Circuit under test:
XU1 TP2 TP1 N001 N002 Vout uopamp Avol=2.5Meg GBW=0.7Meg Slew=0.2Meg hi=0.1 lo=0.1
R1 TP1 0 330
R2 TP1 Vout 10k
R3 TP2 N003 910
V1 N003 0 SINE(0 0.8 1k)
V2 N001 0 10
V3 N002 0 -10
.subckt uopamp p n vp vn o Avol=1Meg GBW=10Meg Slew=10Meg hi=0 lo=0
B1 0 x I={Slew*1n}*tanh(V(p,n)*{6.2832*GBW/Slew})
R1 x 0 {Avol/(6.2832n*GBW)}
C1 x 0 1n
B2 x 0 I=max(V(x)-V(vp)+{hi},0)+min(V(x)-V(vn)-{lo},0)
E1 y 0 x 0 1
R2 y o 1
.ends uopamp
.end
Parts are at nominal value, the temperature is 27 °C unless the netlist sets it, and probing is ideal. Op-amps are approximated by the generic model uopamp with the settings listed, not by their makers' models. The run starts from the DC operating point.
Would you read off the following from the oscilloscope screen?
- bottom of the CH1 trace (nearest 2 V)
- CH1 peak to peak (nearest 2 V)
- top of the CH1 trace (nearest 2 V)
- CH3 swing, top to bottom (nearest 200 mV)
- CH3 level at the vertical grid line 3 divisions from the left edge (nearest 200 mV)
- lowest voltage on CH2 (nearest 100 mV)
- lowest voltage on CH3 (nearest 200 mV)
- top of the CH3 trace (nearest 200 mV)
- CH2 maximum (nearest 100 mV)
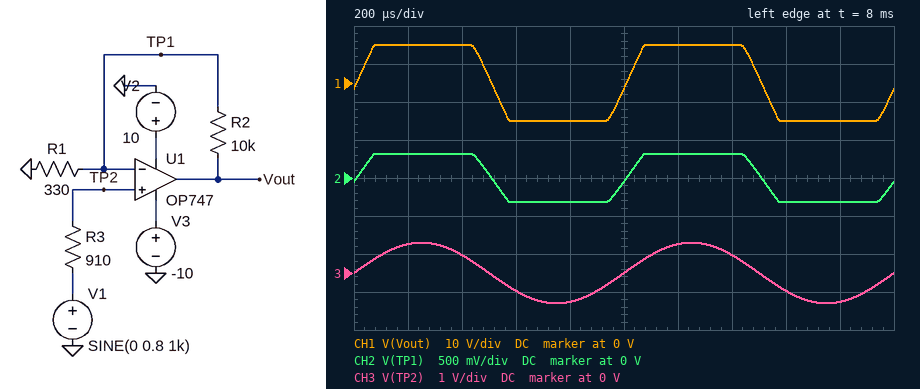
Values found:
-10 V
20 V
10 V
1.6 V
-400 mV
-300 mV
-800 mV
800 mV
300 mV
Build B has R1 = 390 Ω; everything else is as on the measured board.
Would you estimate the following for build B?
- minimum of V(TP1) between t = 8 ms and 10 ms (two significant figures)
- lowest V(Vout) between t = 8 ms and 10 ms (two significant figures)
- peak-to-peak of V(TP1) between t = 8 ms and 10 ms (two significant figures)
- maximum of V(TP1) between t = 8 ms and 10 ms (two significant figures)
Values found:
-370 mV
-9.9 V
740 mV
370 mV
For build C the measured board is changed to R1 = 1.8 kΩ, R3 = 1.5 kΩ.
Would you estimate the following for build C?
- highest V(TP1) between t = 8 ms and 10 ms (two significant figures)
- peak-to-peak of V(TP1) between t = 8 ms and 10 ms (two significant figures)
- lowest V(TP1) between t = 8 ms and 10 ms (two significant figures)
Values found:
800 mV
1.6 V
-800 mV
